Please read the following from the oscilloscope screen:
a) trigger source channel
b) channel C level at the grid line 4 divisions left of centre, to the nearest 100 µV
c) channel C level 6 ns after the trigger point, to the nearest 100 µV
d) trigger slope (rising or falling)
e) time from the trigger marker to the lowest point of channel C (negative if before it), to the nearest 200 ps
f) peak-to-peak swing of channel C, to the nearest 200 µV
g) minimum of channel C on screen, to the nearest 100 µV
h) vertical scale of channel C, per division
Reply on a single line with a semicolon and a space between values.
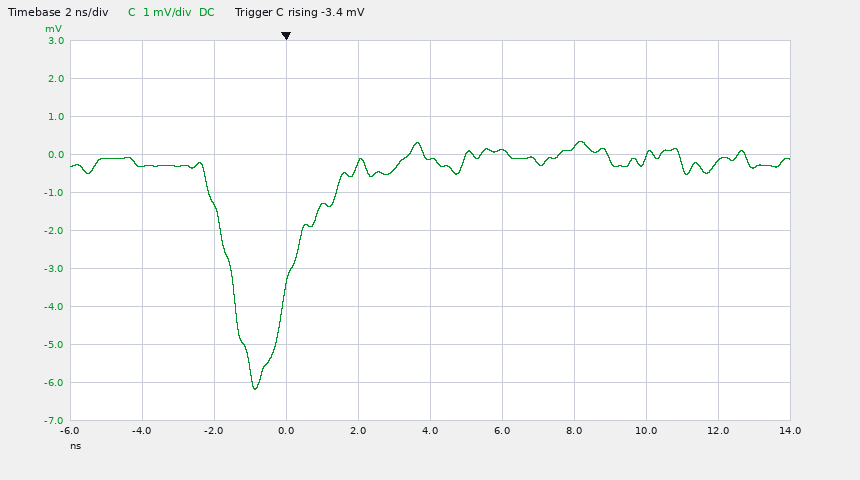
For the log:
channel C; -300 µV; 100 µV; rising; -800 ps; 6.6 mV; -6.2 mV; 1 mV
